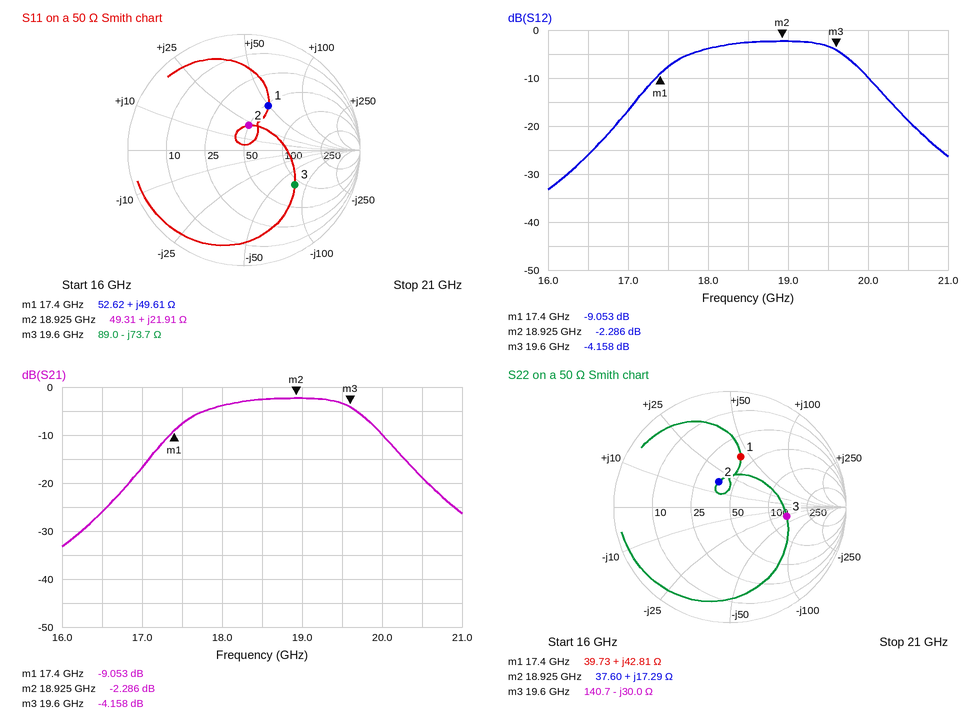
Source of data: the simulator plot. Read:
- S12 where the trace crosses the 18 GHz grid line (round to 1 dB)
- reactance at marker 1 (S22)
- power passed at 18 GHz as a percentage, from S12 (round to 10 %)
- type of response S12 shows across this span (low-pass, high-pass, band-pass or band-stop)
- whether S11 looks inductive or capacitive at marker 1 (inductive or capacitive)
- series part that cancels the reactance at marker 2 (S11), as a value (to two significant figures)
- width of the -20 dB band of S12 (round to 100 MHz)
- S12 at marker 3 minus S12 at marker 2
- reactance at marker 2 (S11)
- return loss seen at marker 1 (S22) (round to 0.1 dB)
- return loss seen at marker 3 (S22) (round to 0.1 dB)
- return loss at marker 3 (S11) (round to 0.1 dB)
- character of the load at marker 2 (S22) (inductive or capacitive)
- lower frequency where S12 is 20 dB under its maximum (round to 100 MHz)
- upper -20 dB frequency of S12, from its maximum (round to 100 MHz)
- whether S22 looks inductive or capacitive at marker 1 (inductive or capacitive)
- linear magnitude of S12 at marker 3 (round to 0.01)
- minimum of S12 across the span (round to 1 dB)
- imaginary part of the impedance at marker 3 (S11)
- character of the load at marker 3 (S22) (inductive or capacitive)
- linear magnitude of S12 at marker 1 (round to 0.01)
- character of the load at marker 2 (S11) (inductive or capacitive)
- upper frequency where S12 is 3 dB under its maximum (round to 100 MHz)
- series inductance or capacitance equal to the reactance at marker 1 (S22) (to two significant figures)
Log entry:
-4 dB
+42.81 Ω
40 %
band-pass
inductive
380 fF
4.0 GHz
-1.872 dB
+21.91 Ω
7.1 dB
6.1 dB
5.5 dB
inductive
16.7 GHz
20.7 GHz
inductive
0.62
-33 dB
-73.7 Ω
capacitive
0.35
inductive
19.7 GHz
390 pH
